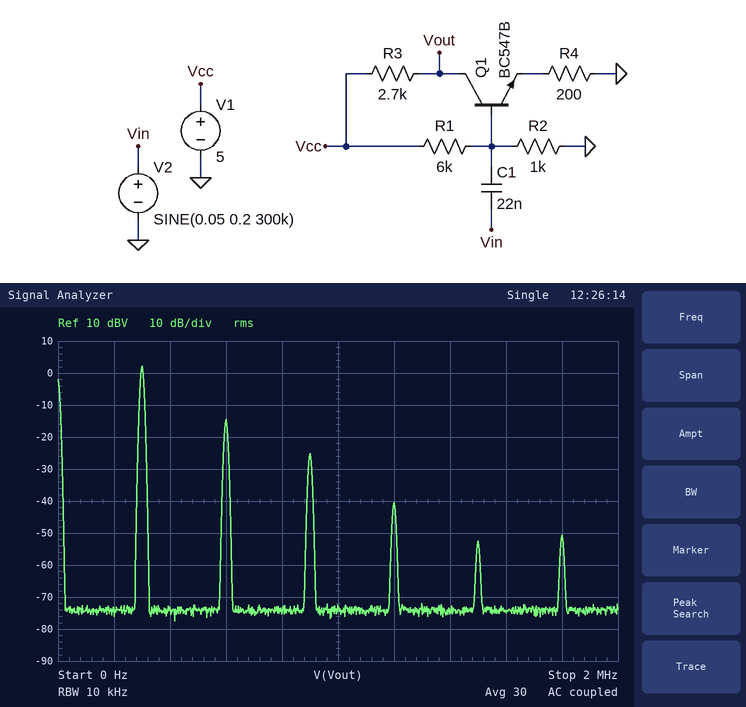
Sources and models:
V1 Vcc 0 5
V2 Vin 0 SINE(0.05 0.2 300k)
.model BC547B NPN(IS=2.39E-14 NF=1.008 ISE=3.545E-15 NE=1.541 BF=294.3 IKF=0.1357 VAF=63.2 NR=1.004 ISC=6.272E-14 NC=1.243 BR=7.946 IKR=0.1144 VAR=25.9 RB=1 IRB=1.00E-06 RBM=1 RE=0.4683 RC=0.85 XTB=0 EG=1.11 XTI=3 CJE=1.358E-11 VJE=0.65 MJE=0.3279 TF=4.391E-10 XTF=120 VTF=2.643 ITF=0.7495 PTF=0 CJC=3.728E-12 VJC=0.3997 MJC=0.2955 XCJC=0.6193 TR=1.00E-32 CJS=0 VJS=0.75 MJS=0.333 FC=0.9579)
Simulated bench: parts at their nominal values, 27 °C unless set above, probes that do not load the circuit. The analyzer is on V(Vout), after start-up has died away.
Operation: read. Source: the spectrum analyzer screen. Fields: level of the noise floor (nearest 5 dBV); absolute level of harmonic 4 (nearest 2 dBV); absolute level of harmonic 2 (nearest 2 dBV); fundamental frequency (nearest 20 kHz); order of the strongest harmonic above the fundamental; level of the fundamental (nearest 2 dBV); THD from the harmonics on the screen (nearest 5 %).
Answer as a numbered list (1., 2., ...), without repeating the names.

1. -75 dBV
2. -40 dBV
3. -14 dBV
4. 300 kHz
5. 2
6. 2 dBV
7. 15 %
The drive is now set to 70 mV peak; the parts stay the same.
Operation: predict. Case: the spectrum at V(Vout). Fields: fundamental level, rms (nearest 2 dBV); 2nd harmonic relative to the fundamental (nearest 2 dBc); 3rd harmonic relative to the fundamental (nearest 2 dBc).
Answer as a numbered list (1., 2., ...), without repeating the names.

1. -6 dBV
2. -30 dBc
3. -48 dBc
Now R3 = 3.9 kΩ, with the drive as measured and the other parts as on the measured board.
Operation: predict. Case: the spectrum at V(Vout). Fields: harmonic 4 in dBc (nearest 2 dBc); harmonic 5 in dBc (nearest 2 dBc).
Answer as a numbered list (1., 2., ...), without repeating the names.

1. -36 dBc
2. -36 dBc
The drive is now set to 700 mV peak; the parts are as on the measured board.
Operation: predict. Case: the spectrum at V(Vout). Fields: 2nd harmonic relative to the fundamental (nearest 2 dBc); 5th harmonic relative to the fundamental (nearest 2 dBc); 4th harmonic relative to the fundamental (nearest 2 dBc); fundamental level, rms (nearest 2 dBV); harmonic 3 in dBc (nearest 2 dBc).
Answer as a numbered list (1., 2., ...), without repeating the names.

1. -10 dBc
2. -28 dBc
3. -14 dBc
4. 6 dBV
5. -16 dBc
